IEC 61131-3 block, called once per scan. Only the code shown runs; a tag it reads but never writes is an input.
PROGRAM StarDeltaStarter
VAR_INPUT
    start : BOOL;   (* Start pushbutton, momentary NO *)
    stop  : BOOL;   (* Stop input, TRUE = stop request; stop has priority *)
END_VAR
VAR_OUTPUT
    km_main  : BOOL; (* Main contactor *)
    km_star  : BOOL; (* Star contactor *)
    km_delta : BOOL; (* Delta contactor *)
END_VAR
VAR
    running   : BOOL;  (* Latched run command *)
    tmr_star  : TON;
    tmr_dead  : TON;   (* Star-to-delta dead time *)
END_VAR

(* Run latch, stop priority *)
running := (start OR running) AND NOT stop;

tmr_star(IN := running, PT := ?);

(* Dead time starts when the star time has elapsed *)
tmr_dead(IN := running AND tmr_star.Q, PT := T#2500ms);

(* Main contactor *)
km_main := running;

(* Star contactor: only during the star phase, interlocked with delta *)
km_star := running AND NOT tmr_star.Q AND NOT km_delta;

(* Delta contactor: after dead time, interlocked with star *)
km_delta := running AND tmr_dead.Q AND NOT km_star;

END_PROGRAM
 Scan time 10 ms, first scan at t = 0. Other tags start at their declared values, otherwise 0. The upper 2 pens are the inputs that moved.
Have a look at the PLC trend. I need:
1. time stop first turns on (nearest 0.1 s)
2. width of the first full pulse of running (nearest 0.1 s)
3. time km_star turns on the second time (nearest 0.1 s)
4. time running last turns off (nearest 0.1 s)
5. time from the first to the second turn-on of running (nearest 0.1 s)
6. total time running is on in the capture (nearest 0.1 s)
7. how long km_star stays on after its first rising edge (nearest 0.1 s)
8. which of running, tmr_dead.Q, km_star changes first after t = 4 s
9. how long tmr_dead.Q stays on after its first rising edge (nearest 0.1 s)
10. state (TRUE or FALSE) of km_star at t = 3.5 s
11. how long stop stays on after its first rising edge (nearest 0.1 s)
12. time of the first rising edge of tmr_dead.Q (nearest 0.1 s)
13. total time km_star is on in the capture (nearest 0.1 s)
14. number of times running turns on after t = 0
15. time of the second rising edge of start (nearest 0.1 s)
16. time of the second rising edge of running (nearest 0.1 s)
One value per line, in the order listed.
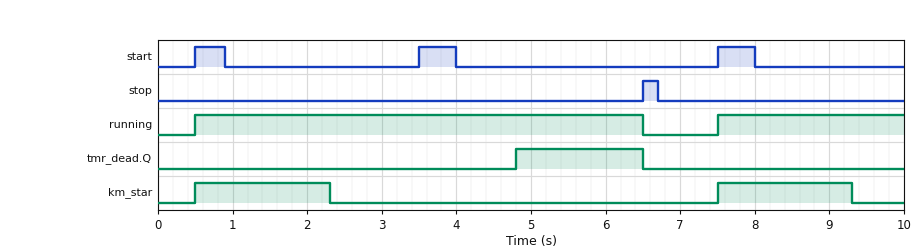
6.5 s
6.0 s
7.5 s
6.5 s
7.0 s
8.5 s
1.8 s
tmr_dead.Q
1.7 s
FALSE
0.2 s
4.8 s
3.6 s
2
3.5 s
7.5 s
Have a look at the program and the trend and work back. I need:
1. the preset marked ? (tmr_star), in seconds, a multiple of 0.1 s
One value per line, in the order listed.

1.8 s
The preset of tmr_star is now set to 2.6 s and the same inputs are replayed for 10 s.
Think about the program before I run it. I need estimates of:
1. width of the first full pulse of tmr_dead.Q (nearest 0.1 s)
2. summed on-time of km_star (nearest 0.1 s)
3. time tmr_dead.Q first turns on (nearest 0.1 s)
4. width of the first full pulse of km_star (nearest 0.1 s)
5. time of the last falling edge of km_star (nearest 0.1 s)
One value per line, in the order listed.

0.9 s
5.1 s
5.6 s
2.6 s
3.1 s
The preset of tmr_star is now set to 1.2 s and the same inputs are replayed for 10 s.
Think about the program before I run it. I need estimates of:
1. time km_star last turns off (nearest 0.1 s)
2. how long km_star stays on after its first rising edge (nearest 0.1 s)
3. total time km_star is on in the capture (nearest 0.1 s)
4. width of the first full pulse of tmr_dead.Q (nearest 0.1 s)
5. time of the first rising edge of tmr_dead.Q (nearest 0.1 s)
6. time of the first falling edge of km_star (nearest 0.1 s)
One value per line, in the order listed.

8.7 s
1.2 s
2.4 s
2.3 s
4.2 s
1.7 s
